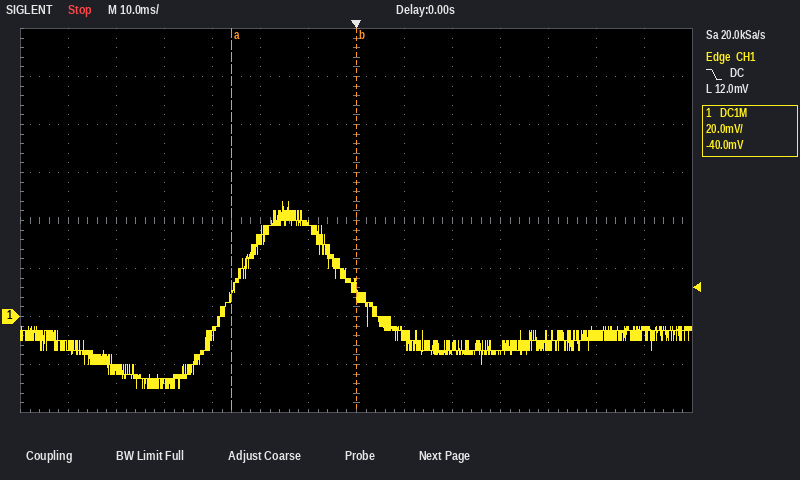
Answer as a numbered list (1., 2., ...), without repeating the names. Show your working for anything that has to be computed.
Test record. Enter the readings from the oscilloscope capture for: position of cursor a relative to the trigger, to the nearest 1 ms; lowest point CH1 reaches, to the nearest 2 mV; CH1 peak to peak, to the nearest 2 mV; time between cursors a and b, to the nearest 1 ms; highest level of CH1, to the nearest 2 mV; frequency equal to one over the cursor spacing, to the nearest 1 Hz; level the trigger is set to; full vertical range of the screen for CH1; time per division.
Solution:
1. -26 ms
2. -30 mV
3. 48 mV − (-30 mV) = 78 mV
4. 26 ms
5. 48 mV
6. 1 / 26 ms ≈ 38 Hz
7. 12.0 mV
8. 160 mV
9. 10 ms
